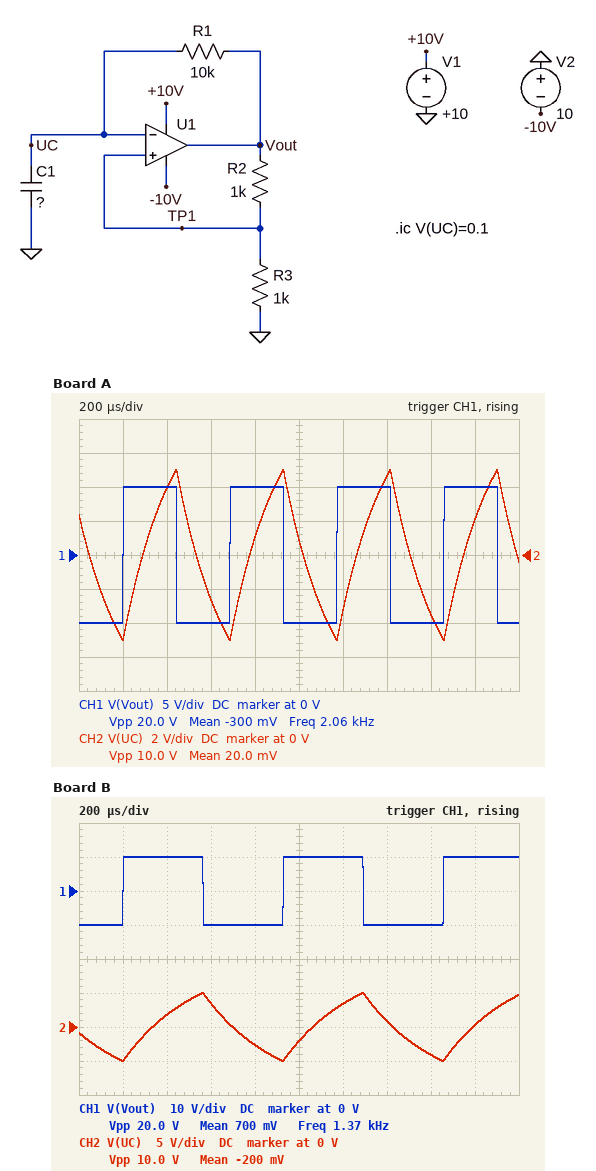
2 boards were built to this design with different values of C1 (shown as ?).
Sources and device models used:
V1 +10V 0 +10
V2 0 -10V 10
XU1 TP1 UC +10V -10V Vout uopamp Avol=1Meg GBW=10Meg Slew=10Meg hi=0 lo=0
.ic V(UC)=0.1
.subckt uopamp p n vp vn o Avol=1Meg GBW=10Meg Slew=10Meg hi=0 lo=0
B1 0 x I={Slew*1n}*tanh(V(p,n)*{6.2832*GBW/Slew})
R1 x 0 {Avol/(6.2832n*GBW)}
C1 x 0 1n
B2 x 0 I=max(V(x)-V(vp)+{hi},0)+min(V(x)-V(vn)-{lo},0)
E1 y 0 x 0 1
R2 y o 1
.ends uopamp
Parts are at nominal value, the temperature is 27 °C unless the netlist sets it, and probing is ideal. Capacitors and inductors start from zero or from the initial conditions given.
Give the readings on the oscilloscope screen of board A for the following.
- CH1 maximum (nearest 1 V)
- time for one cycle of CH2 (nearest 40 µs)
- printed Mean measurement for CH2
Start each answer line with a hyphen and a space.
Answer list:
- 10 V
- 480 µs
- 20.0 mV
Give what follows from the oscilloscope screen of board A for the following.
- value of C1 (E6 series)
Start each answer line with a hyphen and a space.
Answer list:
- 22 nF
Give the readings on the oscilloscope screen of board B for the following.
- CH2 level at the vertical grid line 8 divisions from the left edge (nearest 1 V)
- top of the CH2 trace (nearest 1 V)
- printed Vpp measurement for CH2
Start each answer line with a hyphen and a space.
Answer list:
- -4 V
- 5 V
- 10.0 V
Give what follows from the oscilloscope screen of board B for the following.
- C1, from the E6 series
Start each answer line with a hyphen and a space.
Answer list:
- 33 nF
